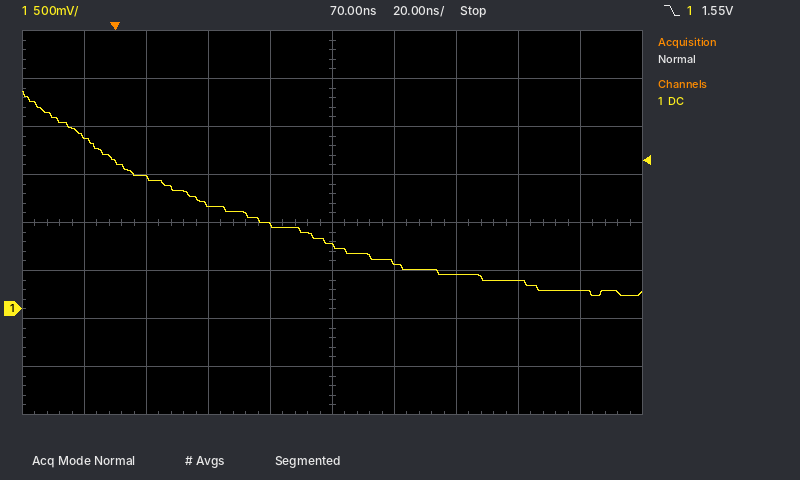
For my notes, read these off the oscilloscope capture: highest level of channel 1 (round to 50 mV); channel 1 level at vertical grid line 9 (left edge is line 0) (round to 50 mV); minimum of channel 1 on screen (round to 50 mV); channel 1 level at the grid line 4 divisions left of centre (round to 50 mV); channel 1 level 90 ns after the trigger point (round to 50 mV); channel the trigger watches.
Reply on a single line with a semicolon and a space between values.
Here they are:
2.25 V; 200 mV; 150 mV; 1.80 V; 500 mV; channel 1
